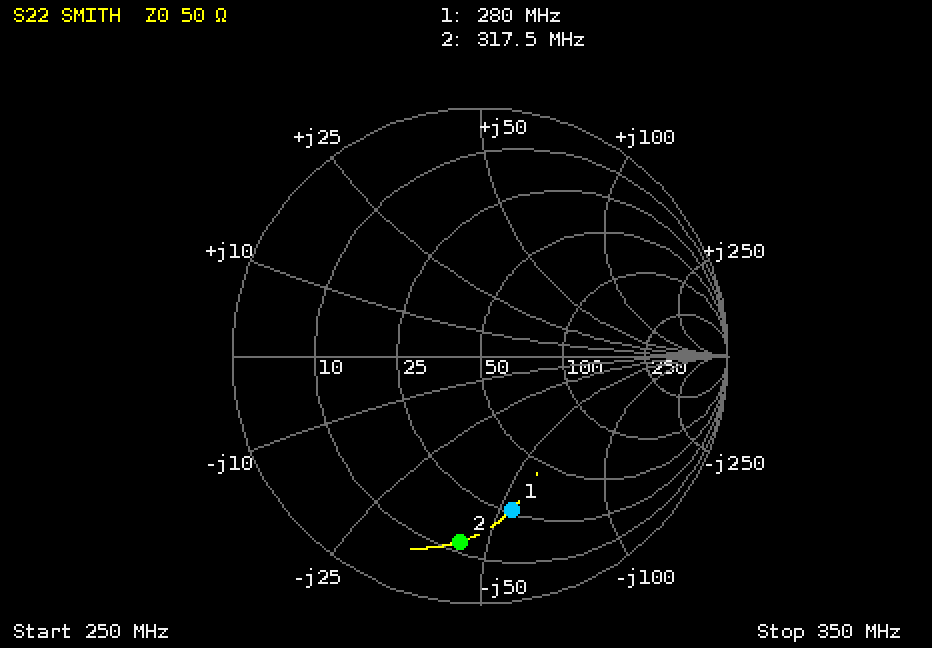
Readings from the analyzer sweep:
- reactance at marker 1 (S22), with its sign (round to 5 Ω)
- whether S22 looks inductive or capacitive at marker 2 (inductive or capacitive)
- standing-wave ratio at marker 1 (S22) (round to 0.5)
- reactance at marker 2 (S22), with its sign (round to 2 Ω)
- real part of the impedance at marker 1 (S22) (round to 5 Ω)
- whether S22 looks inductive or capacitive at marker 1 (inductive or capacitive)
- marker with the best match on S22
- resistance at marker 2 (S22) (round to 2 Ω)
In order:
-55 Ω
capacitive
4.5
-44 Ω
25 Ω
capacitive
marker 1
12 Ω
